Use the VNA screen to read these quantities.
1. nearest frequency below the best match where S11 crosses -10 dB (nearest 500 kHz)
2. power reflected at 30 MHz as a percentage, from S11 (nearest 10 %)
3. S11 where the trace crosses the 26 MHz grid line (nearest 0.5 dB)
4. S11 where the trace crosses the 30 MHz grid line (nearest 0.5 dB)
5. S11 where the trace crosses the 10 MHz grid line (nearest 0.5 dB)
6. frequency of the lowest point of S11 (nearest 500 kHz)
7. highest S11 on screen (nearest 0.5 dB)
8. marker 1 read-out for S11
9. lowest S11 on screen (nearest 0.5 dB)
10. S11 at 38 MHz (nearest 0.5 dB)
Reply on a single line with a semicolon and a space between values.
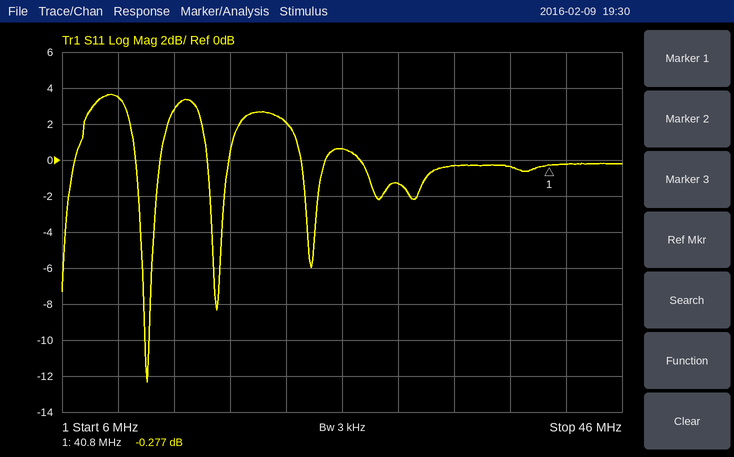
12.0 MHz; 70 %; 0.5 dB; -1.5 dB; 3.5 dB; 12.0 MHz; 3.5 dB; -0.277 dB; -12.5 dB; -0.5 dB
